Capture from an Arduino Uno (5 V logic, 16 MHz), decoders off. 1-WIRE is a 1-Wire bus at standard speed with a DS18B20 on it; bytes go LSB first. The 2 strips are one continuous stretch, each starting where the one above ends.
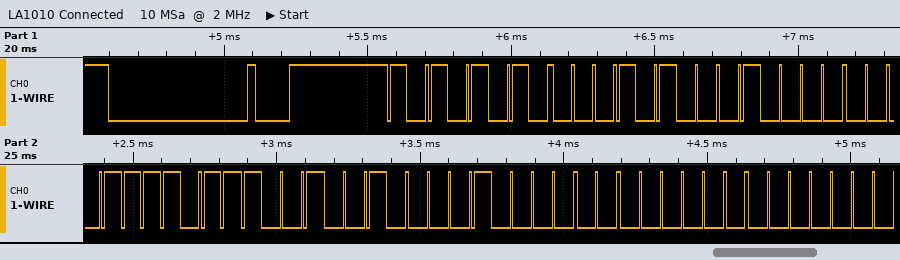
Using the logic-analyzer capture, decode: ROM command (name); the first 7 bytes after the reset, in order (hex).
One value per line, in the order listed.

Match ROM
55 28 02 DE 49 08 00
